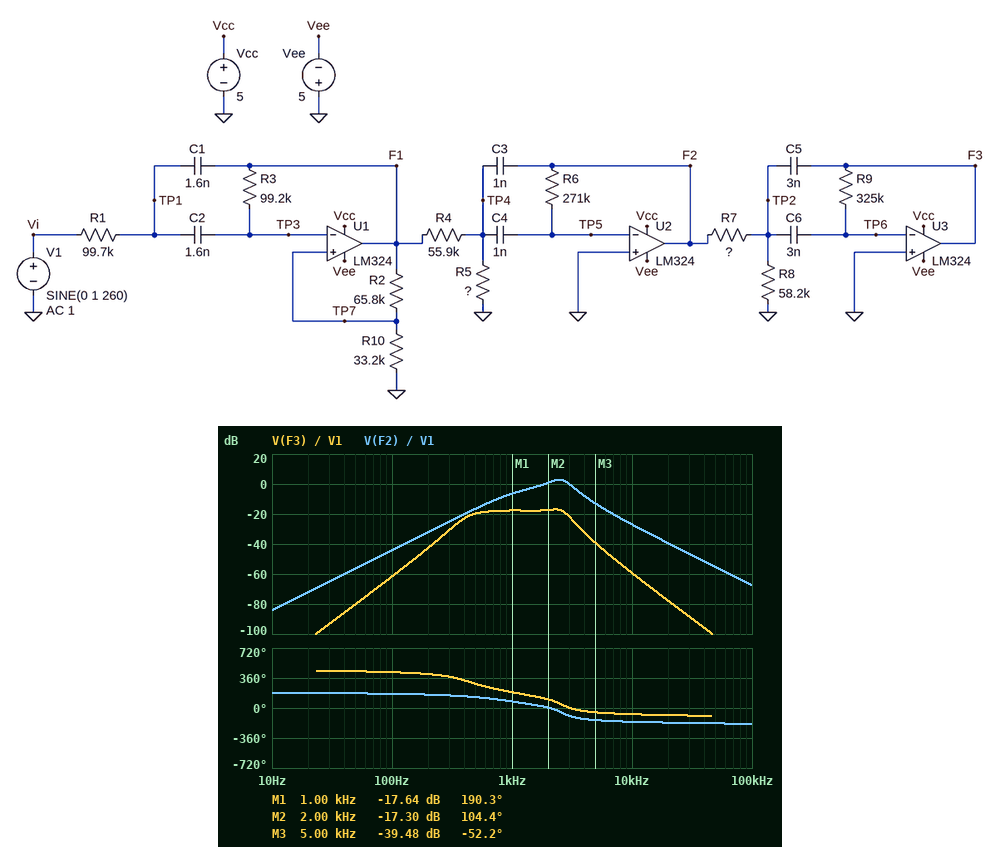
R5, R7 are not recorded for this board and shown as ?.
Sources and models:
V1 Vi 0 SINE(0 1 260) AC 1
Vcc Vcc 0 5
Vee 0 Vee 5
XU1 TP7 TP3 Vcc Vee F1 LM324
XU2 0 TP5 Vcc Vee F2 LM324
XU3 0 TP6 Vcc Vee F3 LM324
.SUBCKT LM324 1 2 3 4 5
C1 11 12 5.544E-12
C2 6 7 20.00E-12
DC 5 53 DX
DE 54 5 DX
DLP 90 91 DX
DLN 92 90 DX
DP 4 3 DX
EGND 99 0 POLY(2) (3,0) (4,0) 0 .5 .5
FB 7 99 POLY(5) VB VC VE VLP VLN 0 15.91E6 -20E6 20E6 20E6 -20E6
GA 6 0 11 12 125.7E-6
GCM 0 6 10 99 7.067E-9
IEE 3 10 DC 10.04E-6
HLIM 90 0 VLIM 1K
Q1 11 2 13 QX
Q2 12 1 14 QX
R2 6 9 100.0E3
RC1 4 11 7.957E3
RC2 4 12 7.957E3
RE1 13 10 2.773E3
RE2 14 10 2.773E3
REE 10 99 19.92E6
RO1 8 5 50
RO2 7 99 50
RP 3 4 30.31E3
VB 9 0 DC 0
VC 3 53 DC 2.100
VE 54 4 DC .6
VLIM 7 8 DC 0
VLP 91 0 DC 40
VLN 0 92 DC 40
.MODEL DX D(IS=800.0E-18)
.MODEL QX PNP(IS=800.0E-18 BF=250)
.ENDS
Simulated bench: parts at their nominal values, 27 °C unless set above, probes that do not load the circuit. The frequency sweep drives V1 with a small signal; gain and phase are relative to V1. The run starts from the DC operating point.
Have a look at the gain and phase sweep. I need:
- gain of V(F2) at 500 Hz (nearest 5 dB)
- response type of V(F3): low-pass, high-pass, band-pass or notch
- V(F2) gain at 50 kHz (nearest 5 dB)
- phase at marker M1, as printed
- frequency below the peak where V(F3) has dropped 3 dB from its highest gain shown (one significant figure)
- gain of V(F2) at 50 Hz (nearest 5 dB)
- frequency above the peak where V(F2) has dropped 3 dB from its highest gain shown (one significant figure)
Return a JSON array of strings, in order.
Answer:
["-15 dB", "band-pass", "-55 dB", "190.3 deg", "500 Hz", "-55 dB", "3 kHz"]
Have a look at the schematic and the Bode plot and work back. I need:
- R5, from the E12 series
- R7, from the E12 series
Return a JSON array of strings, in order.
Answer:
["18 kΩ", "220 kΩ"]
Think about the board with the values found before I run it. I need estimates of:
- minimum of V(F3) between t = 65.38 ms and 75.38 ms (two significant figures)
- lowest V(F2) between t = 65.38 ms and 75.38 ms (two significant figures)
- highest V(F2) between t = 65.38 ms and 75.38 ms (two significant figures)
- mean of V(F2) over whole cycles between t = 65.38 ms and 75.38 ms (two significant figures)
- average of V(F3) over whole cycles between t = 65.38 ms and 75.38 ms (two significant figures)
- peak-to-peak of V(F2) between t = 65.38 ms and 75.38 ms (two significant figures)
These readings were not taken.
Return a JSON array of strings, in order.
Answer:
["-24 mV", "-47 mV", "37 mV", "-5.4 mV", "-6.5 mV", "84 mV"]
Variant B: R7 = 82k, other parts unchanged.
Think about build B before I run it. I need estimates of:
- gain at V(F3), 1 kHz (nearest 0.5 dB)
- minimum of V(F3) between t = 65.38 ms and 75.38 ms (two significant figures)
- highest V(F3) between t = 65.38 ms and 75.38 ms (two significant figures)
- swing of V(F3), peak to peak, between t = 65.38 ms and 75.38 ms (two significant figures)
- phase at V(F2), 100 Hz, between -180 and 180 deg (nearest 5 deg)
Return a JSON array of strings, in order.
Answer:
["-8.5 dB", "-41 mV", "28 mV", "69 mV", "170 deg"]
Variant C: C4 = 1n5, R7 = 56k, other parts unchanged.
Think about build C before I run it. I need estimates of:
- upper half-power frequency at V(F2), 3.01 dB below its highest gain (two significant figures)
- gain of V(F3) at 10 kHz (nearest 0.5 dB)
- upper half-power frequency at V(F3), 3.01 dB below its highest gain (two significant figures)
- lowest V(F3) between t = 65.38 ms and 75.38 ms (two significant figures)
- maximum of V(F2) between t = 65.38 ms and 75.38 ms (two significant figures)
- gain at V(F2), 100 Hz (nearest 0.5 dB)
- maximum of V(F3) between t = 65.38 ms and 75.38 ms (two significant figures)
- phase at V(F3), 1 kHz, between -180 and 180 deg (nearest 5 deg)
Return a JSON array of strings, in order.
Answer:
["2.5 kHz", "-47.5 dB", "2.3 kHz", "-69 mV", "58 mV", "-40.5 dB", "56 mV", "-170 deg"]
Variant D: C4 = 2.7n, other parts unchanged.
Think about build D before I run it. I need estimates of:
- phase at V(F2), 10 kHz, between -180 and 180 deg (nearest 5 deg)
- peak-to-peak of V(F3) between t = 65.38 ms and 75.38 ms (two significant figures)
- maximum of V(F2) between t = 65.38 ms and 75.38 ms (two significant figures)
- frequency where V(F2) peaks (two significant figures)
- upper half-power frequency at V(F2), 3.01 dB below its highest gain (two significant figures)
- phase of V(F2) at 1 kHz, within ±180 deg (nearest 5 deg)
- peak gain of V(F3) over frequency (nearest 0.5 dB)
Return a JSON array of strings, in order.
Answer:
["-170 deg", "98 mV", "110 mV", "1.5 kHz", "1.9 kHz", "60 deg", "-5.5 dB"]
